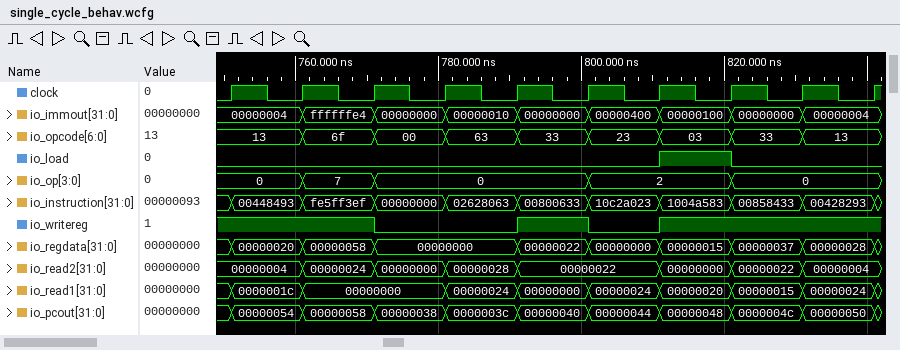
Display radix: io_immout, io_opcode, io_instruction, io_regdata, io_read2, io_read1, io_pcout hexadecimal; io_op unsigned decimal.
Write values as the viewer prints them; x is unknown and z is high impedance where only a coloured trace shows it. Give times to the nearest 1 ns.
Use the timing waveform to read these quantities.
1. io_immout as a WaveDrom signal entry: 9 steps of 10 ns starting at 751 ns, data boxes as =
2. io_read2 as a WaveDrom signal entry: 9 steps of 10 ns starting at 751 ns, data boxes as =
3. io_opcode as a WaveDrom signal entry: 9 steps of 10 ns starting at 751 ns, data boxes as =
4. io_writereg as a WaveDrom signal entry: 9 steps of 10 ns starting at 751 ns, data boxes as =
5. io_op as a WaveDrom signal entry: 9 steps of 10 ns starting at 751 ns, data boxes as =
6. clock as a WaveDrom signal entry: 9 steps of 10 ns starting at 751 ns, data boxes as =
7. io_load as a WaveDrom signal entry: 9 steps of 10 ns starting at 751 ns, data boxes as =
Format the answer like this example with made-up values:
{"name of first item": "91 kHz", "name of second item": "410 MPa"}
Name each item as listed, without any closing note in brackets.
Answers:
{"io_immout as a WaveDrom signal entry: 9 steps of 10 ns starting at 751 ns, data boxes as =": "{name: 'io_immout', wave: '=========', data: '00000004 ffffffe4 00000000 00000010 00000000 00000400 00000100 00000000 00000004'}", "io_read2 as a WaveDrom signal entry: 9 steps of 10 ns starting at 751 ns, data boxes as =": "{name: 'io_read2', wave: '=====.===', data: '00000004 00000024 00000000 00000028 00000022 00000000 00000022 00000004'}", "io_opcode as a WaveDrom signal entry: 9 steps of 10 ns starting at 751 ns, data boxes as =": "{name: 'io_opcode', wave: '=========', data: '13 6f 00 63 33 23 03 33 13'}", "io_writereg as a WaveDrom signal entry: 9 steps of 10 ns starting at 751 ns, data boxes as =": "{name: 'io_writereg', wave: '1.0.101..'}", "io_op as a WaveDrom signal entry: 9 steps of 10 ns starting at 751 ns, data boxes as =": "{name: 'io_op', wave: '===..=.=.', data: '0 7 0 2 0'}", "clock as a WaveDrom signal entry: 9 steps of 10 ns starting at 751 ns, data boxes as =": "{name: 'clock', wave: 'p........'}", "io_load as a WaveDrom signal entry: 9 steps of 10 ns starting at 751 ns, data boxes as =": "{name: 'io_load', wave: '0.....10.'}"}
